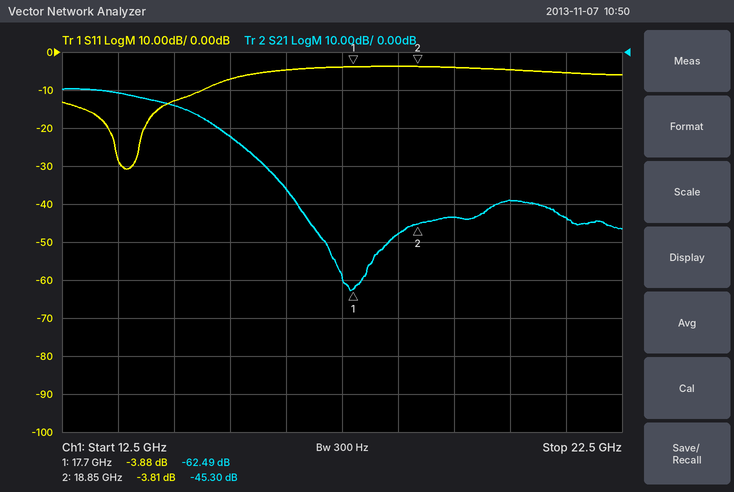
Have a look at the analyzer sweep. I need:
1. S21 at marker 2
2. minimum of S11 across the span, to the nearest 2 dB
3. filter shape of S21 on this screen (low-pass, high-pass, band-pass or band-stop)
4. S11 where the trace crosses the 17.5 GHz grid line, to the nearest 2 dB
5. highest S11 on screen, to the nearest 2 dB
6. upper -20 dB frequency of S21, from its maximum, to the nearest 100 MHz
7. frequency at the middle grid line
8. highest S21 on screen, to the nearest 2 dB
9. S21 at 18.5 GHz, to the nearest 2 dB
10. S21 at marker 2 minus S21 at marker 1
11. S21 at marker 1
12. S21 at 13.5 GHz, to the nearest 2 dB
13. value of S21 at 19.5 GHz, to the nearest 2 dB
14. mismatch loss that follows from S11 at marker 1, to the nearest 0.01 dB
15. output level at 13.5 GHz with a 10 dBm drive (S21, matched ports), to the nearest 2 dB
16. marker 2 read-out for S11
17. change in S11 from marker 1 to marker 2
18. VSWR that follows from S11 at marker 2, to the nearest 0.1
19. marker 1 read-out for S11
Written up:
-45.30 dB
-30 dB
low-pass
-4 dB
-4 dB
16.1 GHz
17.5 GHz
-10 dB
-48 dB
17.19 dB
-62.49 dB
-10 dB
-44 dB
2.29 dB
0 dBm
-3.81 dB
0.07 dB
4.6
-3.88 dB
